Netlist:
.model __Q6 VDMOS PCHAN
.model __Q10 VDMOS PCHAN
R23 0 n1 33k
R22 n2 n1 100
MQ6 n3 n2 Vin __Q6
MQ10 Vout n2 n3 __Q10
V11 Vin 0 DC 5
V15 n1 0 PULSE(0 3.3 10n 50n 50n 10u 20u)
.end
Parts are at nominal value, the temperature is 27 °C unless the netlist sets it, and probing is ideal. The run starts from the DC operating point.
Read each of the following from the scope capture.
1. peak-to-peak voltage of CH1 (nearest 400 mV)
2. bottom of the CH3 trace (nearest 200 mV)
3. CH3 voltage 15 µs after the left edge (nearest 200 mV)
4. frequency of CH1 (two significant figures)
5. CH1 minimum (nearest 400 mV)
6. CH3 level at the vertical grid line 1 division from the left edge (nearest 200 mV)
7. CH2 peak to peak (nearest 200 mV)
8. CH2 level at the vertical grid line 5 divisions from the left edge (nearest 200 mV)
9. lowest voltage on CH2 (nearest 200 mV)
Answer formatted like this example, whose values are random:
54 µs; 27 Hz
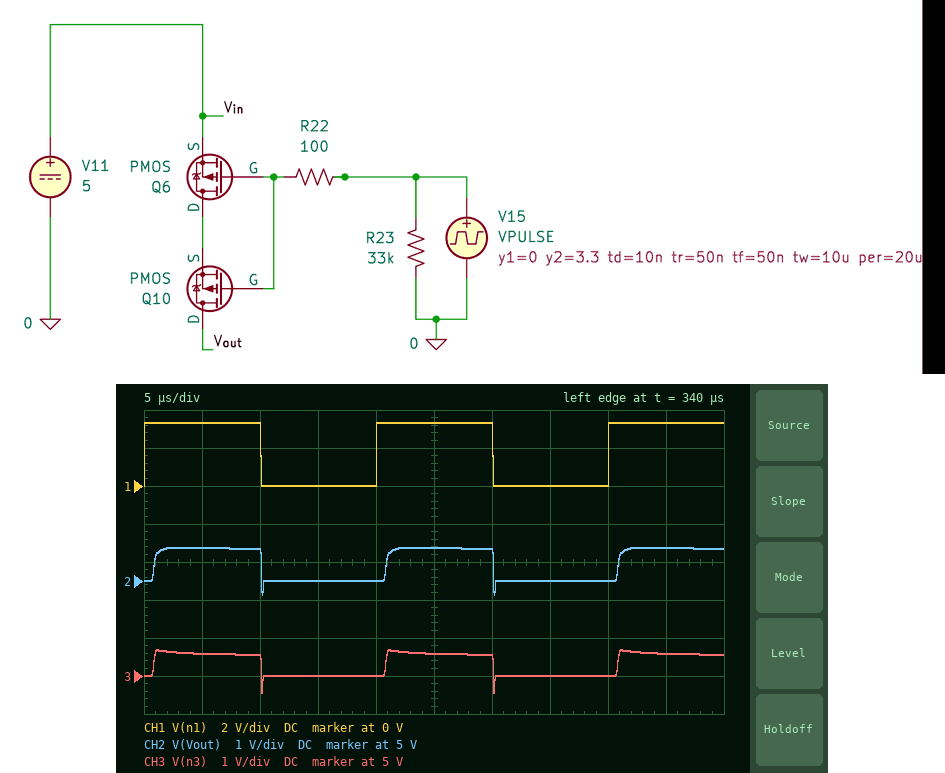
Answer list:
3.2 V; 4.6 V; 5.0 V; 50 kHz; 0 V; 5.6 V; 1.2 V; 5.8 V; 4.6 V
